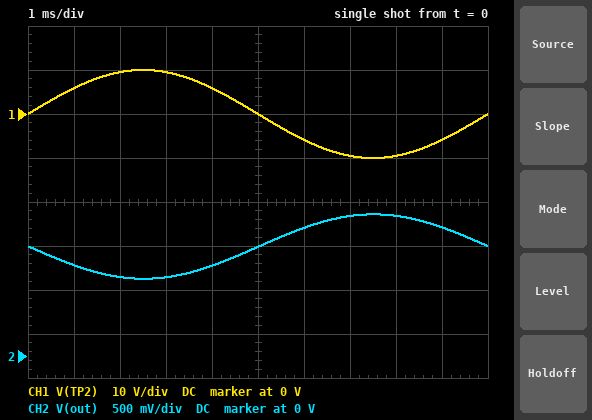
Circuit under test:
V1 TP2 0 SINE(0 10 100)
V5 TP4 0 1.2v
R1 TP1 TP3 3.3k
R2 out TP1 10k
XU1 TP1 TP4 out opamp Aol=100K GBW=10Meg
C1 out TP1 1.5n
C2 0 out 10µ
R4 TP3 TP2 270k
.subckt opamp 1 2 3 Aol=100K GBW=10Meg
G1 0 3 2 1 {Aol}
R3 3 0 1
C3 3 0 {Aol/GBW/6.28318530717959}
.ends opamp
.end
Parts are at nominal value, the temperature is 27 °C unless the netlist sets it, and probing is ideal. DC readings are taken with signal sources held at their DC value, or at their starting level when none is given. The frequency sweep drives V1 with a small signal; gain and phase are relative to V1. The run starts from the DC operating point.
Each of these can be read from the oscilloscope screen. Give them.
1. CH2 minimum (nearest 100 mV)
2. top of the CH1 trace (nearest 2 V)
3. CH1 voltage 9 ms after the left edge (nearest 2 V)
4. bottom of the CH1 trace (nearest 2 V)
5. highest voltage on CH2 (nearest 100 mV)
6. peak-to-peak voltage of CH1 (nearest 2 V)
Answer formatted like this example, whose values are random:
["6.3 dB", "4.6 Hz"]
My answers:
["900 mV", "10 V", "-6 V", "-10 V", "1.6 V", "20 V"]
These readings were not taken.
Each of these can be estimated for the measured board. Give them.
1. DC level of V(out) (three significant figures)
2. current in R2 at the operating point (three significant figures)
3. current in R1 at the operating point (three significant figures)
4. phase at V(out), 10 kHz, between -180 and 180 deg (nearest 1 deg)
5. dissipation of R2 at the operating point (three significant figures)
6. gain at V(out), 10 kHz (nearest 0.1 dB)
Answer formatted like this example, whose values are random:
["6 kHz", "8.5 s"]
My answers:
["1.24 V", "4.39 µA", "4.39 µA", "137 deg", "193 nW", "-31.5 dB"]
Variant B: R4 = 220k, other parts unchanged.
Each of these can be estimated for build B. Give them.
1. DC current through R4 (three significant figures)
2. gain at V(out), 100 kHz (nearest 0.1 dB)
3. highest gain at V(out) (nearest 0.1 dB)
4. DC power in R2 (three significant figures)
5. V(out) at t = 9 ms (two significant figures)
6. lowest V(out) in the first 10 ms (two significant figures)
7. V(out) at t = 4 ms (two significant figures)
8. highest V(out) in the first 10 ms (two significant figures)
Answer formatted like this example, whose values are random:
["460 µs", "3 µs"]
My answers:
["5.37 µA", "-46.5 dB", "-27.0 dB", "289 nW", "1.5 V", "810 mV", "990 mV", "1.7 V"]
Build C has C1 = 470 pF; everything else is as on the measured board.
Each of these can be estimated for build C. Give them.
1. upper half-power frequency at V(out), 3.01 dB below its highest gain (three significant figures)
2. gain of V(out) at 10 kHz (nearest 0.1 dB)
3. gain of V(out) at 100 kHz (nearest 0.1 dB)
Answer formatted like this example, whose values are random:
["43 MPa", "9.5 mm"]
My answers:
["33.9 kHz", "-29.1 dB", "-38.6 dB"]
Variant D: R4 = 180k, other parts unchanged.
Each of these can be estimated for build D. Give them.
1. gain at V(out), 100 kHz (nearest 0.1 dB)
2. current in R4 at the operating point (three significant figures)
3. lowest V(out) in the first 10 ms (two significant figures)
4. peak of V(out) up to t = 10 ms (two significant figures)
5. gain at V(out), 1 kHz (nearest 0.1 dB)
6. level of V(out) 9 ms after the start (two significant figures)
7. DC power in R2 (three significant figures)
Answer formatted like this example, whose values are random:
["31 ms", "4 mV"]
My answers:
["-44.8 dB", "6.55 µA", "720 mV", "1.8 V", "-25.3 dB", "1.6 V", "429 nW"]
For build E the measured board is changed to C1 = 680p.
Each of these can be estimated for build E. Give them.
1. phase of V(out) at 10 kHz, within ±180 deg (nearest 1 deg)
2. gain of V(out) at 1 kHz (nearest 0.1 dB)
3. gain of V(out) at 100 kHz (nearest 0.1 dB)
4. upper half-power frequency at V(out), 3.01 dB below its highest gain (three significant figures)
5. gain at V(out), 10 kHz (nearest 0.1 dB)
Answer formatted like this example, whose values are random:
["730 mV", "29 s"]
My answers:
["157 deg", "-28.7 dB", "-41.6 dB", "23.4 kHz", "-29.5 dB"]
